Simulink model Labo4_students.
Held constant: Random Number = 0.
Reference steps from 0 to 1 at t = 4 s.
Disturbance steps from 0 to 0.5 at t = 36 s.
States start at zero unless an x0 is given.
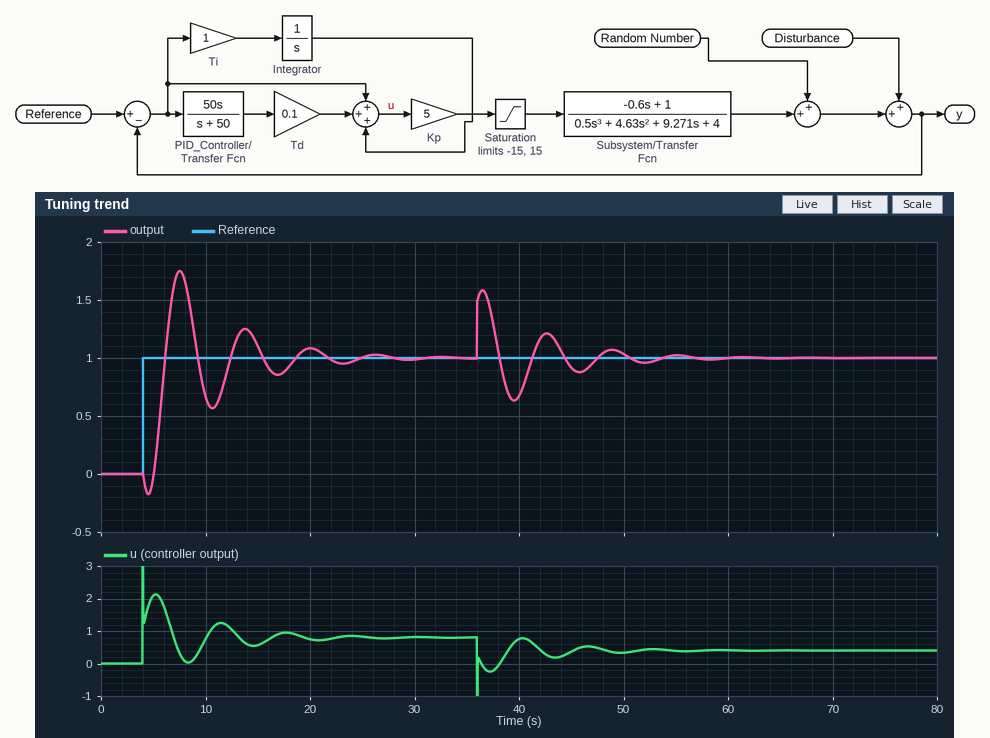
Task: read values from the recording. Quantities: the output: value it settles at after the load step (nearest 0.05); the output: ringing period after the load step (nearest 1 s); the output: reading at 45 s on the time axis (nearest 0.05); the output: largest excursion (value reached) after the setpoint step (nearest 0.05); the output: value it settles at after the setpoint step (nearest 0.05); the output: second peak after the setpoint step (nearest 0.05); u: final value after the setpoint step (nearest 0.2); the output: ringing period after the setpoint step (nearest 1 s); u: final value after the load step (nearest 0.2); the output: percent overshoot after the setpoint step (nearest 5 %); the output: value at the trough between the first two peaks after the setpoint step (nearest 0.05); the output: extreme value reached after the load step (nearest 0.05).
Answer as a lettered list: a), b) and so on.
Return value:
a) 1.00
b) 6 s
c) 0.90
d) 1.75
e) 1.00
f) 1.25
g) 0.8
h) 6 s
i) 0.4
j) 75 %
k) 0.55
l) 1.60
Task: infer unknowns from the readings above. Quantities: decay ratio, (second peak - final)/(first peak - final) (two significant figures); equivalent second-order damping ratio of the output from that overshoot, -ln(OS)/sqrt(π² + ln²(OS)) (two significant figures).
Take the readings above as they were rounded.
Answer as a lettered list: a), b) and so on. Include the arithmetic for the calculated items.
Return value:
a) (1.25 - 1) / (1.75 - 1) = 0.33
b) ln(0.75) = -0.288; 0.288 / sqrt(9.870 + 0.083) = 0.091
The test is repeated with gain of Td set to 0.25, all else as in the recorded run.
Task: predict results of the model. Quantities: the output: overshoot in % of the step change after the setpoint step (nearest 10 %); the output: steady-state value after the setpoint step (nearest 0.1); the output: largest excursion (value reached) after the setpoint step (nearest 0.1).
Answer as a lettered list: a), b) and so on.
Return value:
a) 60 %
b) 1.0
c) 1.6
